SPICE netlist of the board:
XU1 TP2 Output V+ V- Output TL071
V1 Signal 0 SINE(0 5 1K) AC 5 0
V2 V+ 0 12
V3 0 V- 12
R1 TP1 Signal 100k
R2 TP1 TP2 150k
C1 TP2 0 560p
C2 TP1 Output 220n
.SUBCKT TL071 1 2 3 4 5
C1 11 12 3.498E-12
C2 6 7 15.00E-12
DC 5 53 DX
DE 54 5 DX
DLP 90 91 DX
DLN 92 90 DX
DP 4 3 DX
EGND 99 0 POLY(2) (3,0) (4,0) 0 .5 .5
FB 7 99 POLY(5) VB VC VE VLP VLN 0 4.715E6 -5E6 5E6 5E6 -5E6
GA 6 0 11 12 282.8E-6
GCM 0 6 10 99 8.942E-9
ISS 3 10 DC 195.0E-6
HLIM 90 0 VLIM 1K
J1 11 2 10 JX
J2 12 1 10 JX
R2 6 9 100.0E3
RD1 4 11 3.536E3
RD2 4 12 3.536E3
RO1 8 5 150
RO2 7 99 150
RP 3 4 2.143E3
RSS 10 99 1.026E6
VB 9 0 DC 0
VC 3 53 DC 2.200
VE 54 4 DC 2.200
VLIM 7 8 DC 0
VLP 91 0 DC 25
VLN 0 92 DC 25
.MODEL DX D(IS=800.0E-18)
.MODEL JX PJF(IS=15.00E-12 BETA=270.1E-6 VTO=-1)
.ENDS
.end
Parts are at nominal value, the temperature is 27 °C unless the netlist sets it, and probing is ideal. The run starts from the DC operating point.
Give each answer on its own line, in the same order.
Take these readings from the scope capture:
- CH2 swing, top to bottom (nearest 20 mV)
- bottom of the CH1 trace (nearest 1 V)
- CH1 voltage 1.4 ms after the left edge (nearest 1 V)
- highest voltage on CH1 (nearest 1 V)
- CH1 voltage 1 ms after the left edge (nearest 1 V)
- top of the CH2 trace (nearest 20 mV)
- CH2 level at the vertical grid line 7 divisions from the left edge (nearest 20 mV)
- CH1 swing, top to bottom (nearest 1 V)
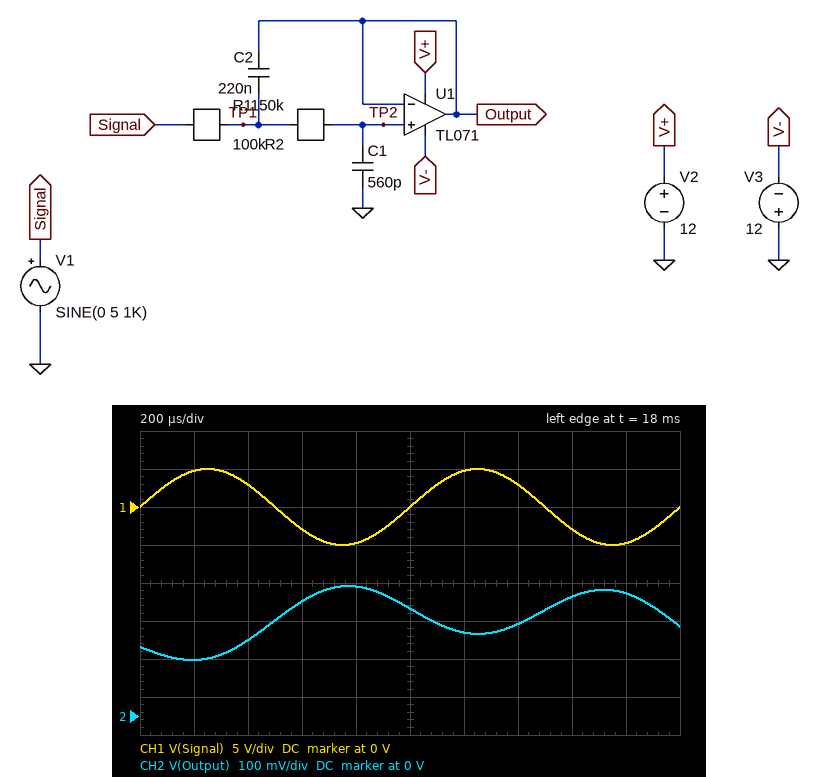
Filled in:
200 mV
-5 V
3 V
5 V
0 V
340 mV
240 mV
10 V
